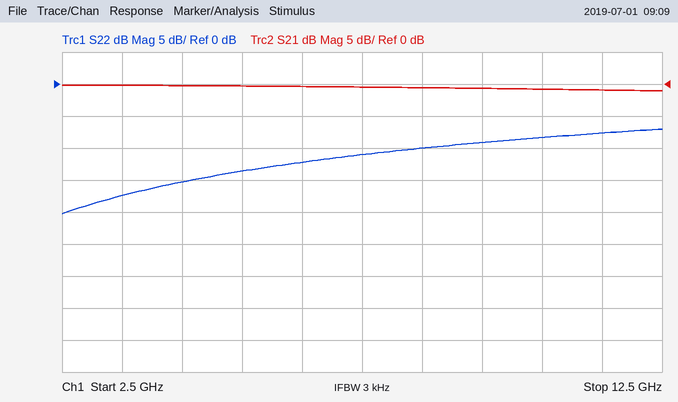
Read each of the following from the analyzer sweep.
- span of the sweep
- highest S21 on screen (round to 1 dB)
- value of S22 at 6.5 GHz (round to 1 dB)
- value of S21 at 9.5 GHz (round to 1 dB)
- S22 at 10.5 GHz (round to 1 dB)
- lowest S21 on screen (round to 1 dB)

10 GHz
0 dB
-12 dB
-1 dB
-8 dB
-1 dB
